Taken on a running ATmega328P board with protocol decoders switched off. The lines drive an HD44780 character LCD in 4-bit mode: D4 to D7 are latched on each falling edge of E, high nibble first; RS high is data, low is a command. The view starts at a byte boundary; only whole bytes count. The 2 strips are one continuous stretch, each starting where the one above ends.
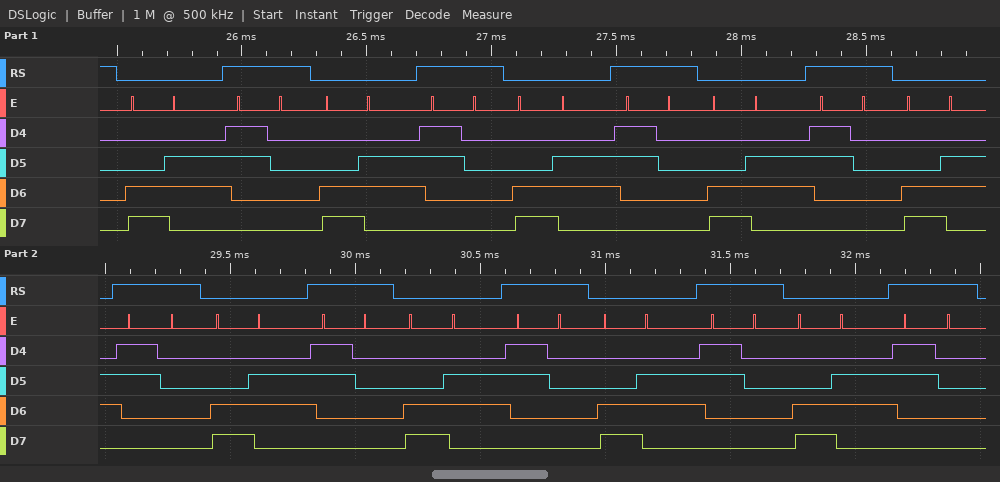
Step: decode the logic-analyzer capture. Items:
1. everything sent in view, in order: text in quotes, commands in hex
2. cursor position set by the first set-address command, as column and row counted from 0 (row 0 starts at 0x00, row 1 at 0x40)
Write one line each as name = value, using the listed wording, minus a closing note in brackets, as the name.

everything sent in view, in order: text in quotes, commands in hex = 0xC6 "0" 0xC6 "0" 0xC6 "0" 0xC6 "0" 0xC6 "0" 0xC6 "0" 0xC6 "0" 0xC6 "0" 0xC6 "0"
cursor position set by the first set-address command, as column and row counted from 0 = column 6, row 1
